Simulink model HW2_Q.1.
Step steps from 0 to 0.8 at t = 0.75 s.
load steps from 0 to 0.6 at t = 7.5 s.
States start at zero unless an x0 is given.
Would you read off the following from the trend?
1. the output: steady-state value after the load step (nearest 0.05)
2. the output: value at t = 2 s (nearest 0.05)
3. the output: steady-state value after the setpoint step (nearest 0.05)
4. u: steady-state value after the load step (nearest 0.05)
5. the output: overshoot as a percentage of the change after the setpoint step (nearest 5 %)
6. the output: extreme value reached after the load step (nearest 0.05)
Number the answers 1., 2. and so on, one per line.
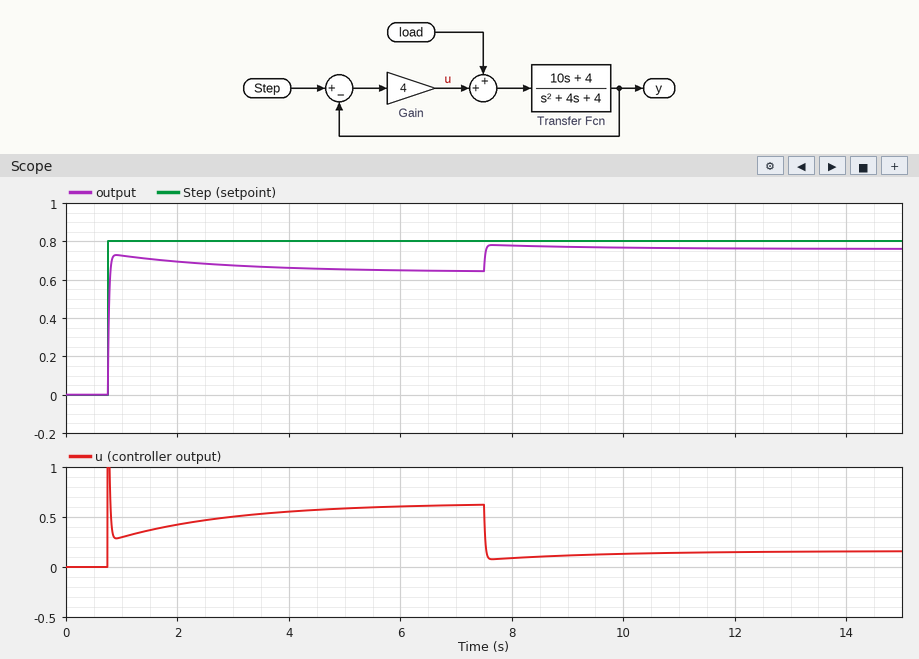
1. 0.75
2. 0.70
3. 0.65
4. 0.15
5. 15 %
6. 0.80
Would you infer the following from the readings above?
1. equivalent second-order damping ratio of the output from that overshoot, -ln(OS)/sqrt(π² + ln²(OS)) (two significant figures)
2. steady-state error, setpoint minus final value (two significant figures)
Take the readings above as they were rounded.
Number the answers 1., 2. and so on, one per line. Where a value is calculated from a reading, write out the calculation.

1. ln(0.15) = -1.897; 1.897 / sqrt(9.870 + 3.599) = 0.52
2. 0.8 - 0.65 = 0.15
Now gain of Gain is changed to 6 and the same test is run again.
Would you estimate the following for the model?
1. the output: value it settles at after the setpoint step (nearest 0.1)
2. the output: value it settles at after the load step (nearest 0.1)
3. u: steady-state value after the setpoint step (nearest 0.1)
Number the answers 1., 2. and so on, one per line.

1. 0.7
2. 0.8
3. 0.7
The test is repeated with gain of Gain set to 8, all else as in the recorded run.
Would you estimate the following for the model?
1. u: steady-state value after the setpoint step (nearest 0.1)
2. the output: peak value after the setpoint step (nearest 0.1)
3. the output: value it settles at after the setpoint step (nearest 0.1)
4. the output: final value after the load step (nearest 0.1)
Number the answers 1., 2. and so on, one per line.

1. 0.7
2. 0.8
3. 0.7
4. 0.8
